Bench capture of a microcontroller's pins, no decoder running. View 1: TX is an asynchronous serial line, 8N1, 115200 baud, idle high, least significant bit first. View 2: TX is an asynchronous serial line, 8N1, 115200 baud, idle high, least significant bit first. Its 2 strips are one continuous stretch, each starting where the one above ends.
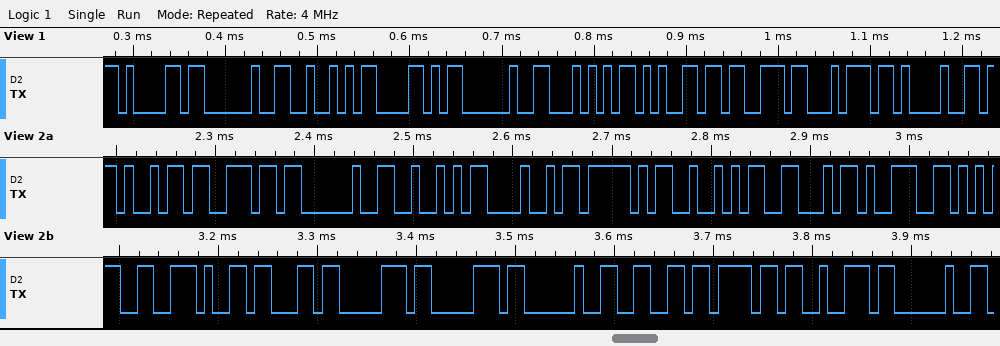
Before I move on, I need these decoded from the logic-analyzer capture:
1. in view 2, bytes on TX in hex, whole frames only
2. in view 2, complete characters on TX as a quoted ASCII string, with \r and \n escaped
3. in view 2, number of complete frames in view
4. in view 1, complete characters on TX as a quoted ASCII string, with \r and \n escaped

69 6E 20 52 48 5F 52 46 39 35 2E 63 70 70 20 66 6F 72 20
"in RH_RF95.cpp for "
19
"a RX Test!"
